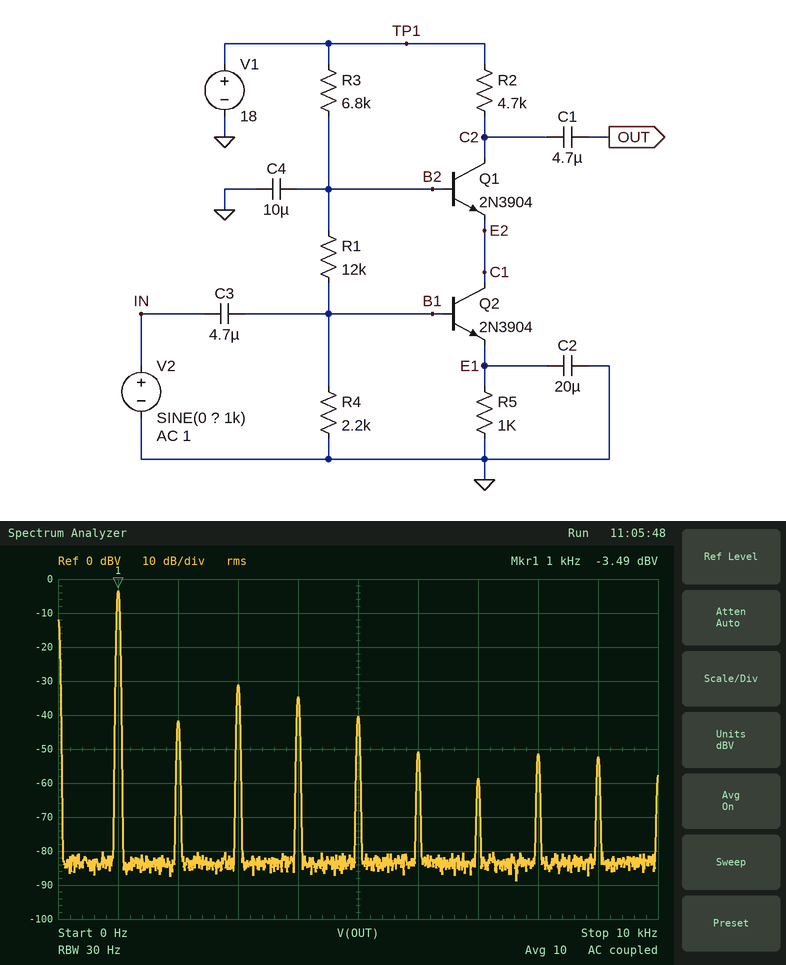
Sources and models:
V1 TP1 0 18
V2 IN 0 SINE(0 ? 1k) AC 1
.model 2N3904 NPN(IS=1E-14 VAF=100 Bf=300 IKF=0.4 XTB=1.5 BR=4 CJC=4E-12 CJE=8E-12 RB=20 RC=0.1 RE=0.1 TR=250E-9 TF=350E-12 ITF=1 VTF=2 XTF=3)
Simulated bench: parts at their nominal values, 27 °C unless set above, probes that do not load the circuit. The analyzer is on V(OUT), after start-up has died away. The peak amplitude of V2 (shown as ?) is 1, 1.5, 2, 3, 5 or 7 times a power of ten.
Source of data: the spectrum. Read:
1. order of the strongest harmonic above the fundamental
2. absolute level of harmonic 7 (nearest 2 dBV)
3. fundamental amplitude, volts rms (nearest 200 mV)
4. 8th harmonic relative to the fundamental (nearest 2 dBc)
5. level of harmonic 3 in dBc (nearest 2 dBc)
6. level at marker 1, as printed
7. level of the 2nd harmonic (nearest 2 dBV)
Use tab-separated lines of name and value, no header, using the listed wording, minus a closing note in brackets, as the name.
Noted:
order of the strongest harmonic above the fundamental	3
absolute level of harmonic 7	-58 dBV
fundamental amplitude, volts rms	600 mV
8th harmonic relative to the fundamental	-48 dBc
level of harmonic 3 in dBc	-28 dBc
level at marker 1, as printed	-3.49 dBV
level of the 2nd harmonic	-42 dBV
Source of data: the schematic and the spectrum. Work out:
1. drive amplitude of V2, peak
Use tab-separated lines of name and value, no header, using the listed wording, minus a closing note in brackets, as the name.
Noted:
drive amplitude of V2, peak	5 mV
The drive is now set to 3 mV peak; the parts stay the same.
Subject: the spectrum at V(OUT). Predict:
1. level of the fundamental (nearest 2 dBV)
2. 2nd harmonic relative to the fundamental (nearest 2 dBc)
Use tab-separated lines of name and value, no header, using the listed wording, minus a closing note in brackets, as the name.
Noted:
level of the fundamental	-8 dBV
2nd harmonic relative to the fundamental	-32 dBc
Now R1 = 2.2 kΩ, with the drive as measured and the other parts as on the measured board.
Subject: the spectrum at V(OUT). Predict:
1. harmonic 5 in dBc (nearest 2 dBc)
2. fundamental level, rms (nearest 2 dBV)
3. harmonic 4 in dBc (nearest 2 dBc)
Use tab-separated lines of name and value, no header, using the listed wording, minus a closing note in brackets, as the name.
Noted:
harmonic 5 in dBc	-30 dBc
fundamental level, rms	-6 dBV
harmonic 4 in dBc	-22 dBc
